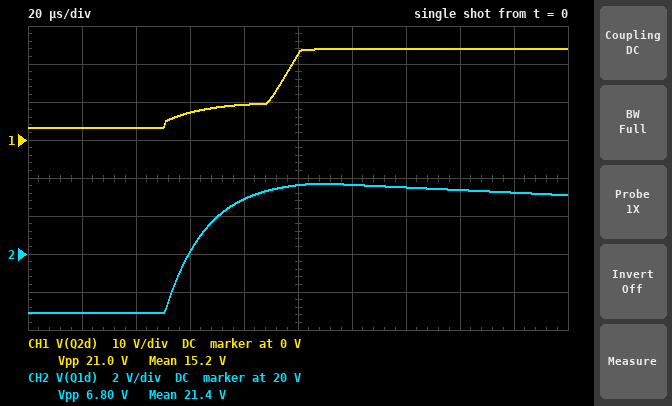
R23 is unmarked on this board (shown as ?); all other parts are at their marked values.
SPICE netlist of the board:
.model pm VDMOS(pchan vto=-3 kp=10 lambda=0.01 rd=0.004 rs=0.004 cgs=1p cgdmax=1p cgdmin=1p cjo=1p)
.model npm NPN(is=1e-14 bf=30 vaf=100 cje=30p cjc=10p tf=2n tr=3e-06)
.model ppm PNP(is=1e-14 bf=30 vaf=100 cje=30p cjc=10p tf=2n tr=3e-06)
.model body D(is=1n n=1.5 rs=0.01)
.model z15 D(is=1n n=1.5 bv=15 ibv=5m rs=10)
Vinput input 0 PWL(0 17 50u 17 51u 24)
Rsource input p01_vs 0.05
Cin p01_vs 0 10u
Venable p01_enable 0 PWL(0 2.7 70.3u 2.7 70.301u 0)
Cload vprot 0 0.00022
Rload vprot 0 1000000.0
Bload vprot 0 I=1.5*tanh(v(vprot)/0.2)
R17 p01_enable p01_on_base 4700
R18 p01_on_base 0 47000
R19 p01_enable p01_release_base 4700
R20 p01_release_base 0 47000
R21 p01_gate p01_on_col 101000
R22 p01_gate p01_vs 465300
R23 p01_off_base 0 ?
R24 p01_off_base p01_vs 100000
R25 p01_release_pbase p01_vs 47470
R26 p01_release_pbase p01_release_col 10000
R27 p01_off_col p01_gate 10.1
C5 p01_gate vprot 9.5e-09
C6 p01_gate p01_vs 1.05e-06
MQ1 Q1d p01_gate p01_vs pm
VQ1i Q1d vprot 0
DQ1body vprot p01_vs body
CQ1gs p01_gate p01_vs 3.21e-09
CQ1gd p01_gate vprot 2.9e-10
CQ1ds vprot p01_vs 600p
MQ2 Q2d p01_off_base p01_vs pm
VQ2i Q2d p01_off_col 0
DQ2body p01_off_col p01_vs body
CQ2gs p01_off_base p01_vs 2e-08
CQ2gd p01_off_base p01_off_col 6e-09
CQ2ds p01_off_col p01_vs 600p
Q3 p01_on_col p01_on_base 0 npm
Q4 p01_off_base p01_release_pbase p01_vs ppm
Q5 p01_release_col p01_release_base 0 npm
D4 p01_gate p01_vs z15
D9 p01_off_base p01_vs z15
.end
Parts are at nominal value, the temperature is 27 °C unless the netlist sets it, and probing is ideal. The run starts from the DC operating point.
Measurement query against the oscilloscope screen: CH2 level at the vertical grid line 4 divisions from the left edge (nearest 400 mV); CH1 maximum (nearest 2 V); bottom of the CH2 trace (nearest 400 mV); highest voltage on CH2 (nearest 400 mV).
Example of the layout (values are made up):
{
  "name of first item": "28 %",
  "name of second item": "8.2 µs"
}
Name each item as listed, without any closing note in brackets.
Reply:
{
  "CH2 level at the vertical grid line 4 divisions from the left edge": "22.8 V",
  "CH1 maximum": "24 V",
  "bottom of the CH2 trace": "16.8 V",
  "highest voltage on CH2": "23.6 V"
}
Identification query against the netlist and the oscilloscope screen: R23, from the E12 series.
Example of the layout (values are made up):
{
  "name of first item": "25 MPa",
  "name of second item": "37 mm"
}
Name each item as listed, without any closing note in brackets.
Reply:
{
  "R23, from the E12 series": "2.7 kΩ"
}
